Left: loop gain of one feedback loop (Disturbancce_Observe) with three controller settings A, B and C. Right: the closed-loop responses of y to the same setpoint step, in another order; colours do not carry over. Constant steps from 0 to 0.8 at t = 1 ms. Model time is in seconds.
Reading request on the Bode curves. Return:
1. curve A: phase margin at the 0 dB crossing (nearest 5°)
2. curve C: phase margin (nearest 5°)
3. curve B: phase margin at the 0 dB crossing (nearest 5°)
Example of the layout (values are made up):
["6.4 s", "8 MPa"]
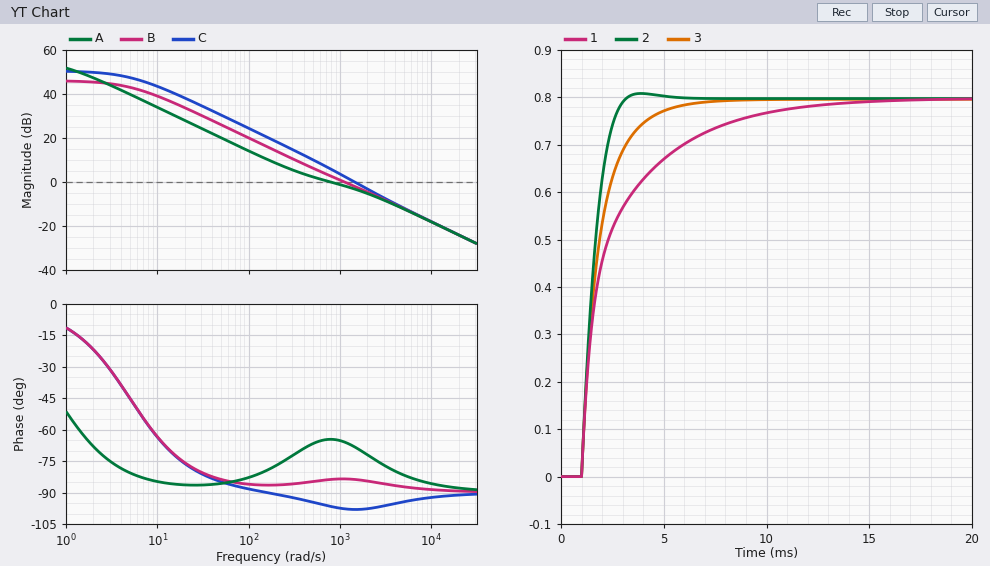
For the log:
["115°", "80°", "95°"]
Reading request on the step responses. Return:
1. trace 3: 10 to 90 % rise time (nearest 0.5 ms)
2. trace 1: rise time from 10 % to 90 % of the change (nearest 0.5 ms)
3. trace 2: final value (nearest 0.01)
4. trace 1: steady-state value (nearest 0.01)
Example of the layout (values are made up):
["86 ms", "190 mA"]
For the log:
["2.5 ms", "5.5 ms", "0.80", "0.80"]
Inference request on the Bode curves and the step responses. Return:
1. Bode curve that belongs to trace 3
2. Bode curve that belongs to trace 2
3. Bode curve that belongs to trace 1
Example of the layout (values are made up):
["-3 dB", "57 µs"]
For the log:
["B", "C", "A"]
